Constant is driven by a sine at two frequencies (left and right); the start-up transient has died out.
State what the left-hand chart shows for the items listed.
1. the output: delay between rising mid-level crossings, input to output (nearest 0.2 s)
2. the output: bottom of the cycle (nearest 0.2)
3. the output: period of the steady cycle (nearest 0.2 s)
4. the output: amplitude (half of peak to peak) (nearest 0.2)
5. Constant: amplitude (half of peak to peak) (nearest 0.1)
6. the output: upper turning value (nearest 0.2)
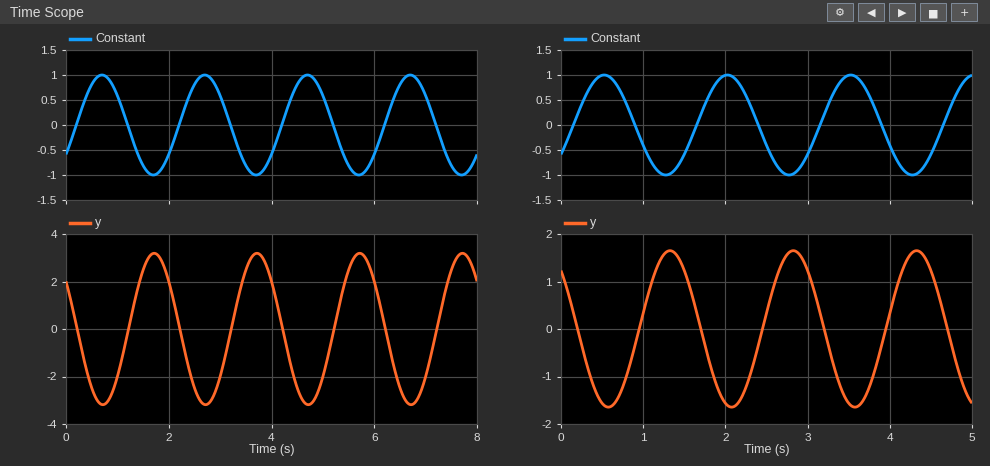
1.0 s
-3.2
2.0 s
3.2
1.0
3.2
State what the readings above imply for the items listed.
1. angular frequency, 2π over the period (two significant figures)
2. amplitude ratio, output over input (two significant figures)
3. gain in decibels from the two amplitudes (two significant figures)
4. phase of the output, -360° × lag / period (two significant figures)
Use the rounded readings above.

3.1 rad/s
3.2
10 dB
-180°
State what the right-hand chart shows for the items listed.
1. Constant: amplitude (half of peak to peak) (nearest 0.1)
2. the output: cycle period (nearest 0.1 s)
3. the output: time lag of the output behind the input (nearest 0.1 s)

1.0
1.5 s
0.8 s
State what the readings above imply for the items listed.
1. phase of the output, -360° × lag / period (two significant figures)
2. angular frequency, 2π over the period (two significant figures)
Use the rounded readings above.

-190°
4.2 rad/s
